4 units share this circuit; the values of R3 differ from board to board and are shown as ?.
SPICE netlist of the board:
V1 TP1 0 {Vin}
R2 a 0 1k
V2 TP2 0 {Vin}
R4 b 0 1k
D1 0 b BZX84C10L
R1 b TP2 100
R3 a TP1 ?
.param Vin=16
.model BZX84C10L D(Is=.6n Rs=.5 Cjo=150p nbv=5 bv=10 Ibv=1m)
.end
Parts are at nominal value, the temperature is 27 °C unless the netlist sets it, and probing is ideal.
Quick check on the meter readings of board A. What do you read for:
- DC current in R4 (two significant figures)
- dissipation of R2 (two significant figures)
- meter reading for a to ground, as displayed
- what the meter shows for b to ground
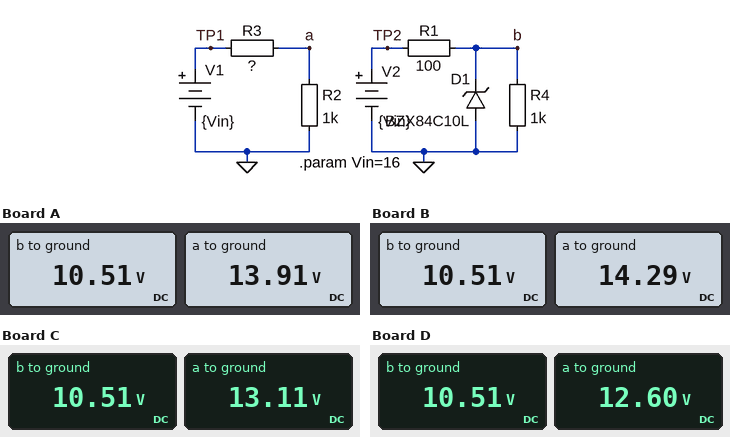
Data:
11 mA
190 mW
13.91 V
10.51 V
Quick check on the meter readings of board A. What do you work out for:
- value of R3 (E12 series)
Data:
150 Ω
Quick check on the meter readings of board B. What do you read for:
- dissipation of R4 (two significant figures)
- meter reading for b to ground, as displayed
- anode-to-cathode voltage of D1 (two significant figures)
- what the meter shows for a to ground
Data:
110 mW
10.51 V
-11 V
14.29 V
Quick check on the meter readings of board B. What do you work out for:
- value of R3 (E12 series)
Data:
120 Ω
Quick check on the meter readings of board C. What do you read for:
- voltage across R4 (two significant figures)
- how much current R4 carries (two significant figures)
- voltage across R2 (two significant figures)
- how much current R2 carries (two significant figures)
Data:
11 V
11 mA
13 V
13 mA
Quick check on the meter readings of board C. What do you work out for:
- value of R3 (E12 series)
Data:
220 Ω
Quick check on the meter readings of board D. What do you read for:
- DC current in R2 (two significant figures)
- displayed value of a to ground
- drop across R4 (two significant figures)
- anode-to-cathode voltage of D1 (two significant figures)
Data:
13 mA
12.60 V
11 V
-11 V
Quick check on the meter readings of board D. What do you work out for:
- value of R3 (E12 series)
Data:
270 Ω
